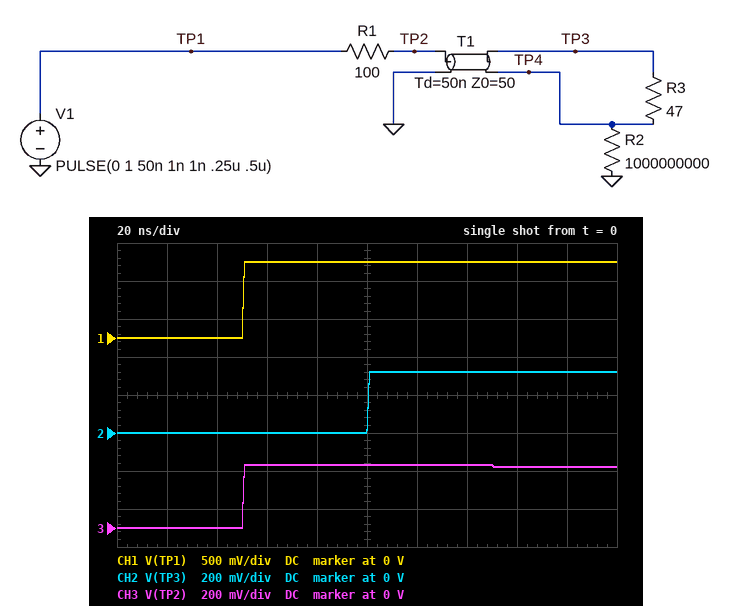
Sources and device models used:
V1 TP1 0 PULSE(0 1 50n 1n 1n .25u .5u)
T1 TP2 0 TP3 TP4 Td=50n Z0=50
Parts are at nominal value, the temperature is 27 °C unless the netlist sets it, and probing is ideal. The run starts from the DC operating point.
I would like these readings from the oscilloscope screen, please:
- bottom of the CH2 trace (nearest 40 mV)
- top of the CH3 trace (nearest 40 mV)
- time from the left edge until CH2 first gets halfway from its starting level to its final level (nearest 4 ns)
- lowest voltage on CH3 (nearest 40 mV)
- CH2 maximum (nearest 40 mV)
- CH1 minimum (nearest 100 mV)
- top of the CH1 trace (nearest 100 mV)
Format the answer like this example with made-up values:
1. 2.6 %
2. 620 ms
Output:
1. 0 V
2. 320 mV
3. 100 ns
4. 0 V
5. 320 mV
6. 0 V
7. 1.0 V
